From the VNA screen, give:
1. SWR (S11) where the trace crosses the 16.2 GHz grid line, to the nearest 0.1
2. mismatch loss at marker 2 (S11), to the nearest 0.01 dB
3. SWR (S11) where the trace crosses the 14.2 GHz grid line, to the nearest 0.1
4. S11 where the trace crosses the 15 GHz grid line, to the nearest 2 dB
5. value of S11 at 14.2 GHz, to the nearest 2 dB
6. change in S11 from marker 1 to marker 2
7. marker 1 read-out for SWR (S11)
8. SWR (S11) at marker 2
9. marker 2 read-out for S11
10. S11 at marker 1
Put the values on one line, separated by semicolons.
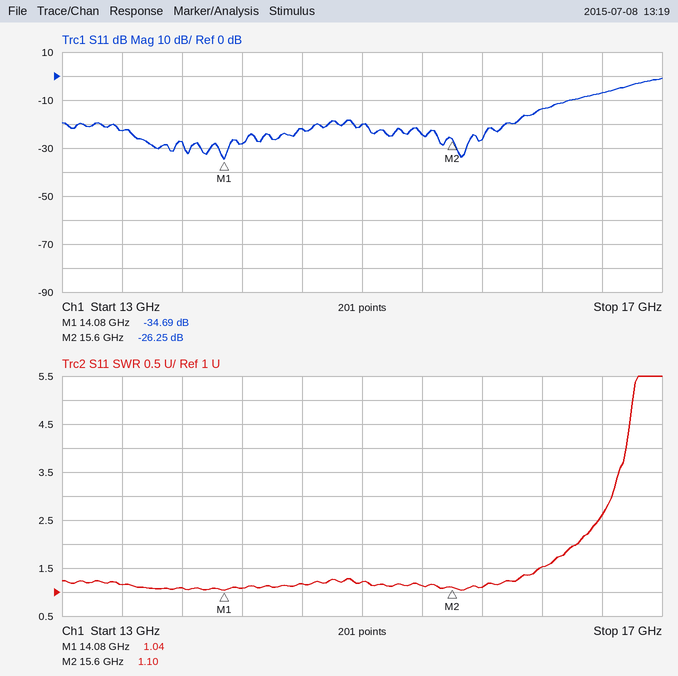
1.5; 0.01 dB; 1.1; -20 dB; -28 dB; 8.44 dB; 1.04; 1.10; -26.25 dB; -34.69 dB
